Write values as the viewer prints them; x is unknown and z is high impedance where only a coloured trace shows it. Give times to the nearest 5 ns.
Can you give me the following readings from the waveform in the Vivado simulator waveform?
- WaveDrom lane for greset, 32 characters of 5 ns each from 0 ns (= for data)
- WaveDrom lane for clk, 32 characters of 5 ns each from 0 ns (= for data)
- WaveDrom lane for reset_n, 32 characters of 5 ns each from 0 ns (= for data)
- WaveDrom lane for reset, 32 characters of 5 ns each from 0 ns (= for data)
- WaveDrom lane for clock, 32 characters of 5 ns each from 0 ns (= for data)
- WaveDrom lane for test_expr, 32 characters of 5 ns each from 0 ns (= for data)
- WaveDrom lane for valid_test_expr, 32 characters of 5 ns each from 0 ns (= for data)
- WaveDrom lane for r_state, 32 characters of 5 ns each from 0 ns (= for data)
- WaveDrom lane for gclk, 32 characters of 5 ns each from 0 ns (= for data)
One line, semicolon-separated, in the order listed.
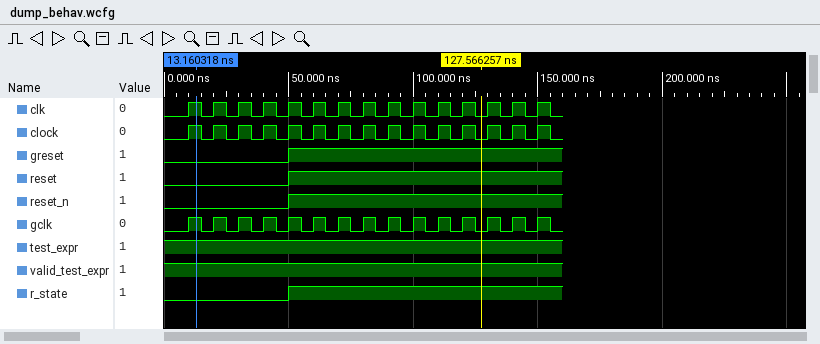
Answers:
{name: 'greset', wave: '0.........1.....................'}; {name: 'clk', wave: '0.101010101010101010101010101010'}; {name: 'reset_n', wave: '0.........1.....................'}; {name: 'reset', wave: '0.........1.....................'}; {name: 'clock', wave: '0.101010101010101010101010101010'}; {name: 'test_expr', wave: '1...............................'}; {name: 'valid_test_expr', wave: '1...............................'}; {name: 'r_state', wave: '0.........1.....................'}; {name: 'gclk', wave: '0.101010101010101010101010101010'}
